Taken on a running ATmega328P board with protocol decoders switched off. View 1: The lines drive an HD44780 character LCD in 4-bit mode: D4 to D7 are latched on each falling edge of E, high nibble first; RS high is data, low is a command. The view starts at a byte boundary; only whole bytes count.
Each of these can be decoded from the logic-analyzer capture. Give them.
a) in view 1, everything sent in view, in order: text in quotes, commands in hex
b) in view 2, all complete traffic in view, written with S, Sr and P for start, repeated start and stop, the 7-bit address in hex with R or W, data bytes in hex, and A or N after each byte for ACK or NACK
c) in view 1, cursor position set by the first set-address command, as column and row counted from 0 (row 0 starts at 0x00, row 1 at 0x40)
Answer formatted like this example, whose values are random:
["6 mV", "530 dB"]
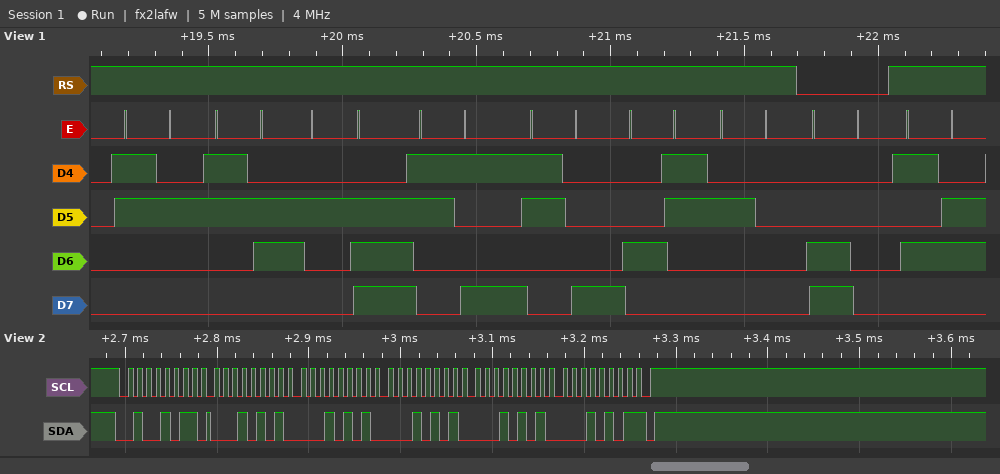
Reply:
["\"26.98C \" 0xC0 \"V\"", "S 25R A 15 A 15 A 15 A 15 A 15 N P", "column 0, row 1"]
